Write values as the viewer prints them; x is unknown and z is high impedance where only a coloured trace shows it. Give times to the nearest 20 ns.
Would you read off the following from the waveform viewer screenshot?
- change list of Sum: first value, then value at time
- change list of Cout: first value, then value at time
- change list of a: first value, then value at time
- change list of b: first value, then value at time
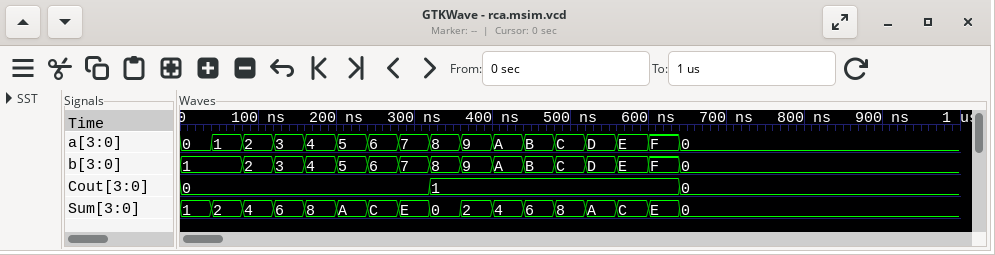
1, 2 at 40 ns, 4 at 80 ns, 6 at 120 ns, 8 at 160 ns, A at 200 ns, C at 240 ns, E at 280 ns, 0 at 320 ns, 2 at 360 ns, 4 at 400 ns, 6 at 440 ns, 8 at 480 ns, A at 520 ns, C at 560 ns, E at 600 ns, 0 at 640 ns
0, 1 at 320 ns, 0 at 640 ns
0, 1 at 40 ns, 2 at 80 ns, 3 at 120 ns, 4 at 160 ns, 5 at 200 ns, 6 at 240 ns, 7 at 280 ns, 8 at 320 ns, 9 at 360 ns, A at 400 ns, B at 440 ns, C at 480 ns, D at 520 ns, E at 560 ns, F at 600 ns, 0 at 640 ns
1, 2 at 80 ns, 3 at 120 ns, 4 at 160 ns, 5 at 200 ns, 6 at 240 ns, 7 at 280 ns, 8 at 320 ns, 9 at 360 ns, A at 400 ns, B at 440 ns, C at 480 ns, D at 520 ns, E at 560 ns, F at 600 ns, 0 at 640 ns
